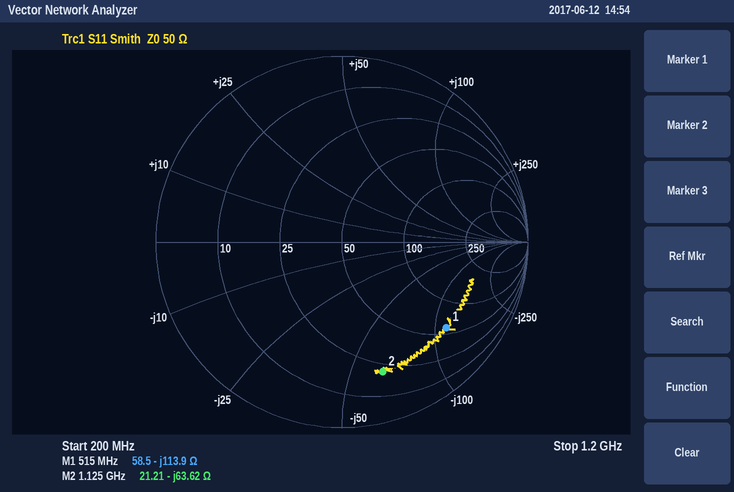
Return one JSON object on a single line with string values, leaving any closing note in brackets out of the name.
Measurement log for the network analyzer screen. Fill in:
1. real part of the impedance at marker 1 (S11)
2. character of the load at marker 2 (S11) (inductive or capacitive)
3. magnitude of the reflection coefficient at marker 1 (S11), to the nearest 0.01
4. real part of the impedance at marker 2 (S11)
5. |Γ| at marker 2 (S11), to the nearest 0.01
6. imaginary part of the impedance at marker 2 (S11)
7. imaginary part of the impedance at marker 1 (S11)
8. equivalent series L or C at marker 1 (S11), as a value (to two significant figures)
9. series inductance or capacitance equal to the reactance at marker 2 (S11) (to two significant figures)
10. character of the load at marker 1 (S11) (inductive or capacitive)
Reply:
{"real part of the impedance at marker 1": "58.5 Ω", "character of the load at marker 2 (S11)": "capacitive", "magnitude of the reflection coefficient at marker 1 (S11), to the nearest 0.01": "0.73", "real part of the impedance at marker 2": "21.21 Ω", "|Γ| at marker 2 (S11), to the nearest 0.01": "0.73", "imaginary part of the impedance at marker 2": "-63.62 Ω", "imaginary part of the impedance at marker 1": "-113.9 Ω", "equivalent series L or C at marker 1 (S11), as a value": "2.7 pF", "series inductance or capacitance equal to the reactance at marker 2 (S11)": "2.2 pF", "character of the load at marker 1 (S11)": "capacitive"}
